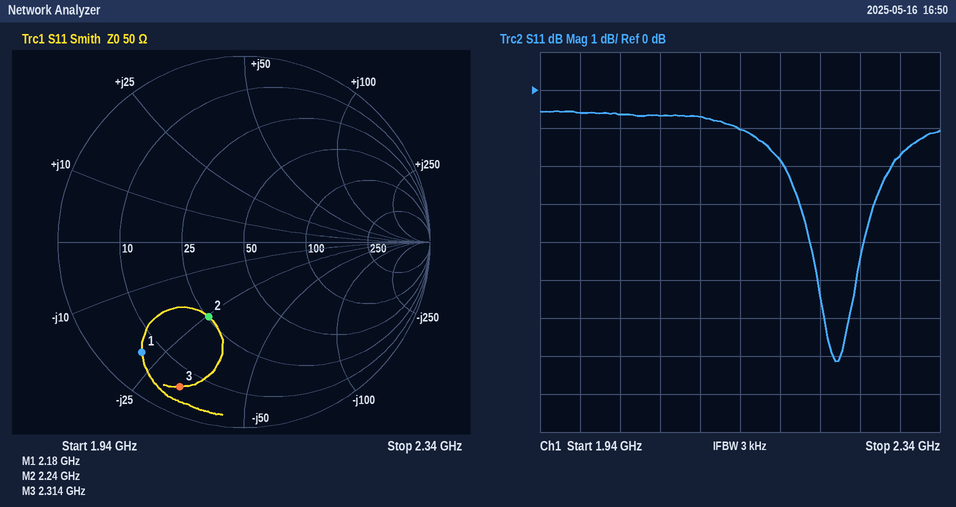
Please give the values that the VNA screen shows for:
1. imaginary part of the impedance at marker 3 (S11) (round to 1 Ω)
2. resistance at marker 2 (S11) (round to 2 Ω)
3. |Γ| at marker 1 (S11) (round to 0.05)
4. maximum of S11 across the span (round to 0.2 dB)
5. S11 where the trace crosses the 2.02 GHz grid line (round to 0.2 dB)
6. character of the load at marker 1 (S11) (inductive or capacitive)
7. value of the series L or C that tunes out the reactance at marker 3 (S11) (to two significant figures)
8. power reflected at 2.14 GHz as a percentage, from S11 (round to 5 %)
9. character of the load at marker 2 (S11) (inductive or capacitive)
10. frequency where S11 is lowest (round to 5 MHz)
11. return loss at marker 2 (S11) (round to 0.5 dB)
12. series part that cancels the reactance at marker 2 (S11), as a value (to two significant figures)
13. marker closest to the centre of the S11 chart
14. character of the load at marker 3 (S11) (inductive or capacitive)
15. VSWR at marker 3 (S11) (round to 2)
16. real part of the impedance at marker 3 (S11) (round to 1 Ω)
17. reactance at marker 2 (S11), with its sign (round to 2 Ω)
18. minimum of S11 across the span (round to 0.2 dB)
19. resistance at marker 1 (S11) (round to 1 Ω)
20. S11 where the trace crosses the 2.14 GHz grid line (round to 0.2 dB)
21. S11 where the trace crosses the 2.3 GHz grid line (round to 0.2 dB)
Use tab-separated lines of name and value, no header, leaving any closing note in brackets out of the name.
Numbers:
imaginary part of the impedance at marker 3 (S11)	-32 Ω
resistance at marker 2 (S11)	26 Ω
|Γ| at marker 1 (S11)	0.80
maximum of S11 across the span	-0.6 dB
S11 where the trace crosses the 2.02 GHz grid line	-0.6 dB
character of the load at marker 1 (S11)	capacitive
value of the series L or C that tunes out the reactance at marker 3 (S11)	2.2 nH
power reflected at 2.14 GHz as a percentage, from S11	80 %
character of the load at marker 2 (S11)	capacitive
frequency where S11 is lowest	2.235 GHz
return loss at marker 2 (S11)	7.0 dB
series part that cancels the reactance at marker 2 (S11), as a value	1.8 nH
marker closest to the centre of the S11 chart	marker 2
character of the load at marker 3 (S11)	capacitive
VSWR at marker 3 (S11)	12
real part of the impedance at marker 3 (S11)	6 Ω
reactance at marker 2 (S11), with its sign	-26 Ω
minimum of S11 across the span	-7.2 dB
resistance at marker 1 (S11)	6 Ω
S11 where the trace crosses the 2.14 GHz grid line	-1.0 dB
S11 where the trace crosses the 2.3 GHz grid line	-1.8 dB
